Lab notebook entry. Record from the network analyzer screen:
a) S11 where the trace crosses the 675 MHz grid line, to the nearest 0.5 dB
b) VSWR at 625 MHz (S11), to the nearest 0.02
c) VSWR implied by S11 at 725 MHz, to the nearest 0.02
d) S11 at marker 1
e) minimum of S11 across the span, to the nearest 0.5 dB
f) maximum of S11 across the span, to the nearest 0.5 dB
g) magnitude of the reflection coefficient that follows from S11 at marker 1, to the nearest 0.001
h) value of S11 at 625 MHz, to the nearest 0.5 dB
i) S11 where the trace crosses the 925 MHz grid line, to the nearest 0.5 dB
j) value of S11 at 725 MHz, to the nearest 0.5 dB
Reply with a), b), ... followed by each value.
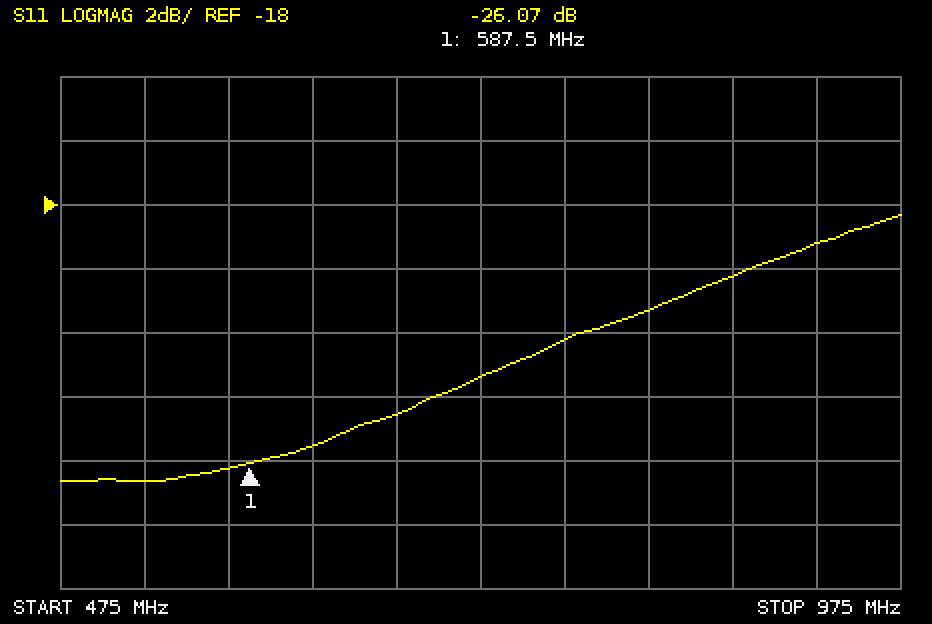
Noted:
a) -24.5 dB
b) 1.12
c) 1.14
d) -26.07 dB
e) -26.5 dB
f) -18.5 dB
g) 0.050
h) -25.5 dB
i) -19.0 dB
j) -23.5 dB
